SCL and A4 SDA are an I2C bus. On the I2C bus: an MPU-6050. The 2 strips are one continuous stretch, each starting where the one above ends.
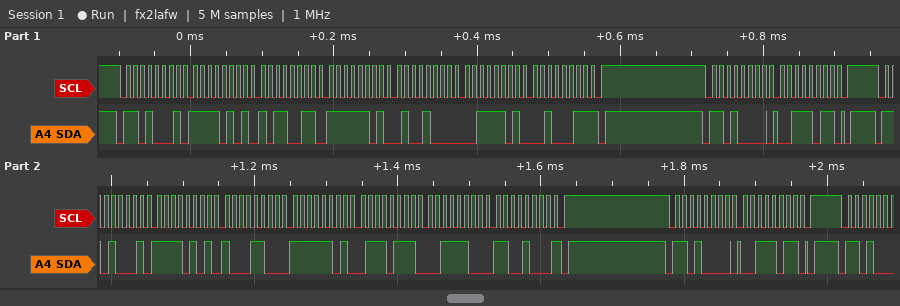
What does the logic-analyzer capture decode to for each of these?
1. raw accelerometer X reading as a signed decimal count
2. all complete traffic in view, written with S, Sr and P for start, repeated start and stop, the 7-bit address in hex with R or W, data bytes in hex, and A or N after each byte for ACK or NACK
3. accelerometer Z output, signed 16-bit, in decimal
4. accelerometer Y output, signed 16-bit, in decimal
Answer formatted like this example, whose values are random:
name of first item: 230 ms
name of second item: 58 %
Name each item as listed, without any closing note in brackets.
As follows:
raw accelerometer X reading as a signed decimal count: -2676
all complete traffic in view, written with S, Sr and P for start, repeated start and stop, the 7-bit address in hex with R or W, data bytes in hex, and A or N after each byte for ACK or NACK: S 68R A F5 A B3 A FD A 48 A 3D A 23 N P S 68W A 3B A P S 68R A F5 A 8C A FD A 77 A 3C A C8 N P S 68W A 3B A P
accelerometer Z output, signed 16-bit, in decimal: 15560
accelerometer Y output, signed 16-bit, in decimal: -649
